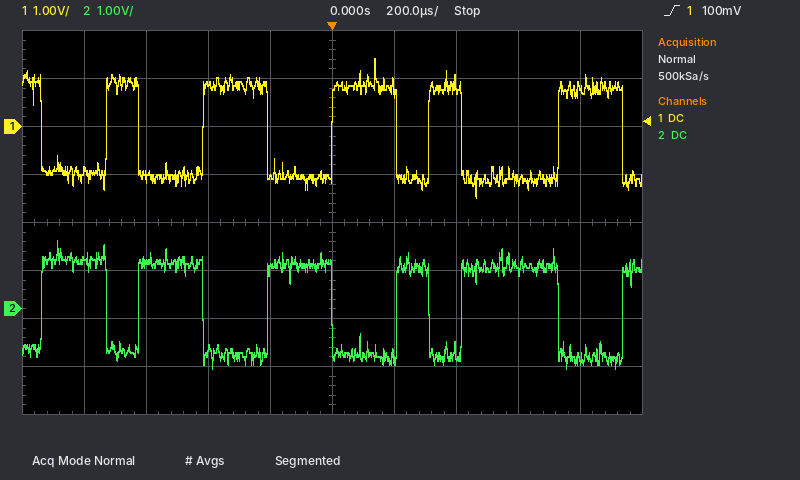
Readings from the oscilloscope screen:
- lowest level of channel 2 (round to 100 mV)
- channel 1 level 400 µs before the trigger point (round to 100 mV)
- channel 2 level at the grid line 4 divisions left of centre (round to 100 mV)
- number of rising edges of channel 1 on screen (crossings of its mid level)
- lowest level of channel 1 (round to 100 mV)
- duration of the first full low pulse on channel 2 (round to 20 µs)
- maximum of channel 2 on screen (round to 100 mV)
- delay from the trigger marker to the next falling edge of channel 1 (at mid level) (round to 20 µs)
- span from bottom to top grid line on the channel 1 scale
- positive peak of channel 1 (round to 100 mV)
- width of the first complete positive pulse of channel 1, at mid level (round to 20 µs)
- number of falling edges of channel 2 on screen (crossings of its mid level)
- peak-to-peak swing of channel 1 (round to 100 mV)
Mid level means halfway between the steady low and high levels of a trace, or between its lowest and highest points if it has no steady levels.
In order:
-1.2 V
900 mV
1.0 V
5
-1.5 V
100 µs
1.4 V
200 µs
8 V
1.4 V
100 µs
5
2.9 V
